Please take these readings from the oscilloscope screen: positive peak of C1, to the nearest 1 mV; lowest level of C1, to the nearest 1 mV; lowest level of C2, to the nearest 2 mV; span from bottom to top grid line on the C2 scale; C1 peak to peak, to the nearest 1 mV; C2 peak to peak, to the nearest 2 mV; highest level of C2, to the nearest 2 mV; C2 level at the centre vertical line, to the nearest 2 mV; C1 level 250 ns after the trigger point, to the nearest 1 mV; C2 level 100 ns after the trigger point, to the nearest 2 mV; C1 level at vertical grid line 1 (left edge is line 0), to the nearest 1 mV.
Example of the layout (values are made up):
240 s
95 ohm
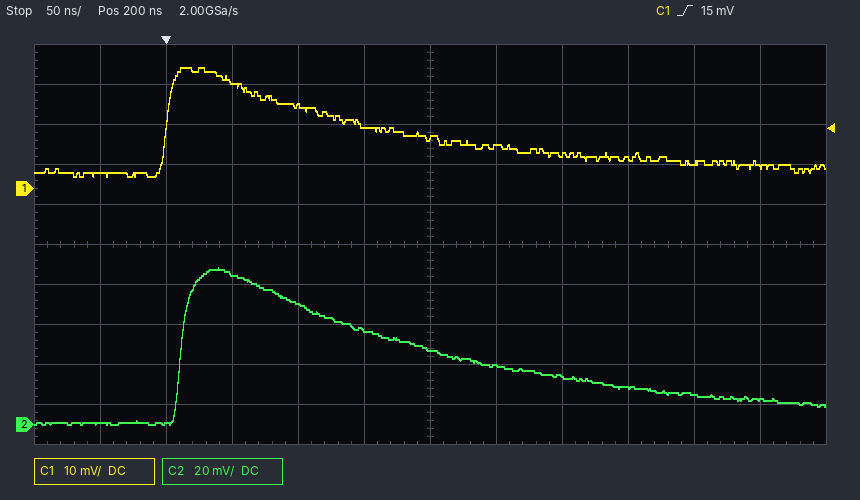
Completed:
30 mV
3 mV
0 mV
200 mV
27 mV
78 mV
78 mV
38 mV
11 mV
60 mV
4 mV
